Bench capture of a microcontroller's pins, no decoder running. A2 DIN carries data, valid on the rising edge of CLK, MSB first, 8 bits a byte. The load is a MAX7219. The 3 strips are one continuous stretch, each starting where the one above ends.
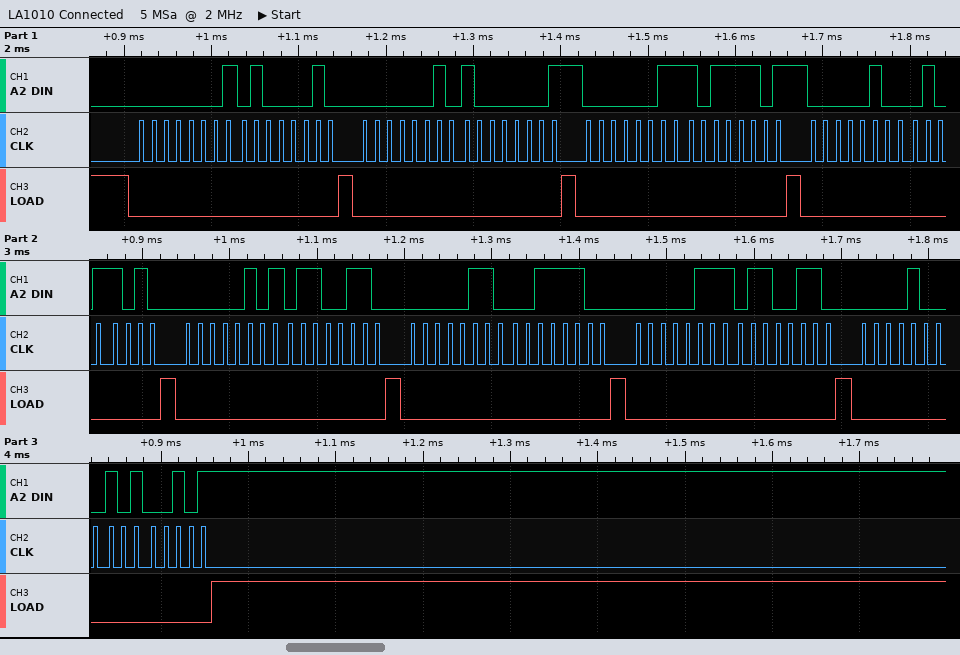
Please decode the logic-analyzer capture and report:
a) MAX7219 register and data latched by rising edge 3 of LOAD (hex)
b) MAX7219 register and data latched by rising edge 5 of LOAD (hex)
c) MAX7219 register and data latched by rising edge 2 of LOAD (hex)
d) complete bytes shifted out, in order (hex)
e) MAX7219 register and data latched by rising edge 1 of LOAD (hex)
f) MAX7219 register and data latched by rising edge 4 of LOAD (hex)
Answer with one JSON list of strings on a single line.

["register 0x3, data 0xBD", "register 0x5, data 0x66", "register 0x2, data 0x81", "01 42 02 81 03 BD 04 5A 05 66 06 3C 07 66 08 A5", "register 0x1, data 0x42", "register 0x4, data 0x5A"]
